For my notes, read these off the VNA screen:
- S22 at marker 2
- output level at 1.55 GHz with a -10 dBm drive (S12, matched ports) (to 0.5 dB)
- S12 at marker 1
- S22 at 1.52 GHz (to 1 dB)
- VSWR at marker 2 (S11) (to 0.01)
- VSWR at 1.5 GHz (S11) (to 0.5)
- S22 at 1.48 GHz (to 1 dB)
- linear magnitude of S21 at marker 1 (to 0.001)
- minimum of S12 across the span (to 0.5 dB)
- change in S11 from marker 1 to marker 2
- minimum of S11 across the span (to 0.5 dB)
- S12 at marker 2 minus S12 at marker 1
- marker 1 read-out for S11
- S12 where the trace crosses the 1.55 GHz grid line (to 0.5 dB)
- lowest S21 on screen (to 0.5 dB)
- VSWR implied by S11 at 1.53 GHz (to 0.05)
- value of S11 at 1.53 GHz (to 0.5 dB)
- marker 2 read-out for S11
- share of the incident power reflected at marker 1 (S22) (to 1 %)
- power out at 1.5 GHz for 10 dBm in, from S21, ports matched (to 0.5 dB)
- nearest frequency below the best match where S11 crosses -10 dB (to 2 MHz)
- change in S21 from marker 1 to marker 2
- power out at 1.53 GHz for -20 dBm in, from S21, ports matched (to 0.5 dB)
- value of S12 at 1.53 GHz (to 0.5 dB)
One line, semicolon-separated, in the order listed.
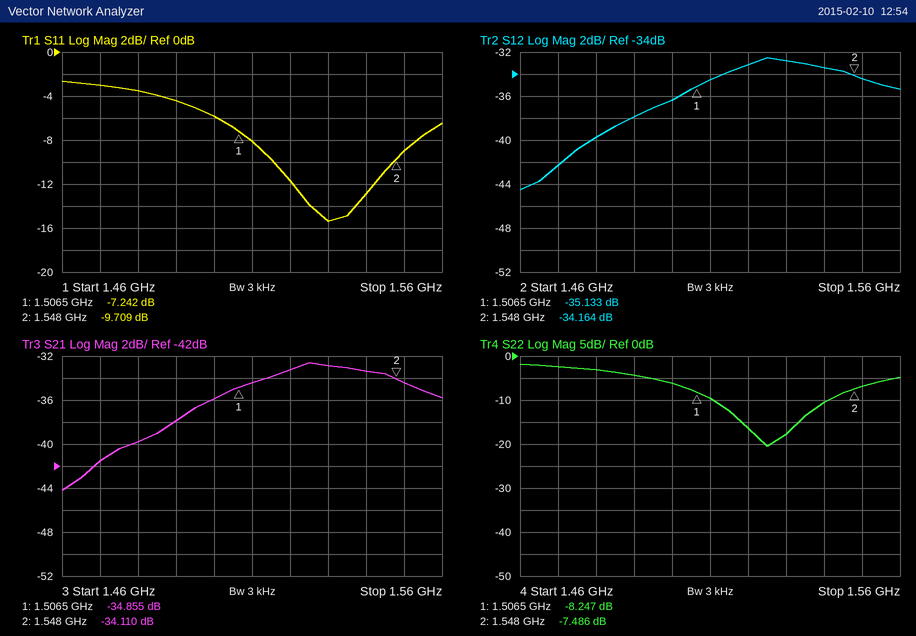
-7.486 dB; -44.5 dBm; -35.133 dB; -16 dB; 1.97; 3.0; -3 dB; 0.018; -44.5 dB; -2.467 dB; -15.5 dB; 0.969 dB; -7.242 dB; -34.5 dB; -44.0 dB; 1.40; -15.5 dB; -9.709 dB; 15 %; -26.0 dBm; 1.516 GHz; 0.745 dB; -53.0 dBm; -33.0 dB
